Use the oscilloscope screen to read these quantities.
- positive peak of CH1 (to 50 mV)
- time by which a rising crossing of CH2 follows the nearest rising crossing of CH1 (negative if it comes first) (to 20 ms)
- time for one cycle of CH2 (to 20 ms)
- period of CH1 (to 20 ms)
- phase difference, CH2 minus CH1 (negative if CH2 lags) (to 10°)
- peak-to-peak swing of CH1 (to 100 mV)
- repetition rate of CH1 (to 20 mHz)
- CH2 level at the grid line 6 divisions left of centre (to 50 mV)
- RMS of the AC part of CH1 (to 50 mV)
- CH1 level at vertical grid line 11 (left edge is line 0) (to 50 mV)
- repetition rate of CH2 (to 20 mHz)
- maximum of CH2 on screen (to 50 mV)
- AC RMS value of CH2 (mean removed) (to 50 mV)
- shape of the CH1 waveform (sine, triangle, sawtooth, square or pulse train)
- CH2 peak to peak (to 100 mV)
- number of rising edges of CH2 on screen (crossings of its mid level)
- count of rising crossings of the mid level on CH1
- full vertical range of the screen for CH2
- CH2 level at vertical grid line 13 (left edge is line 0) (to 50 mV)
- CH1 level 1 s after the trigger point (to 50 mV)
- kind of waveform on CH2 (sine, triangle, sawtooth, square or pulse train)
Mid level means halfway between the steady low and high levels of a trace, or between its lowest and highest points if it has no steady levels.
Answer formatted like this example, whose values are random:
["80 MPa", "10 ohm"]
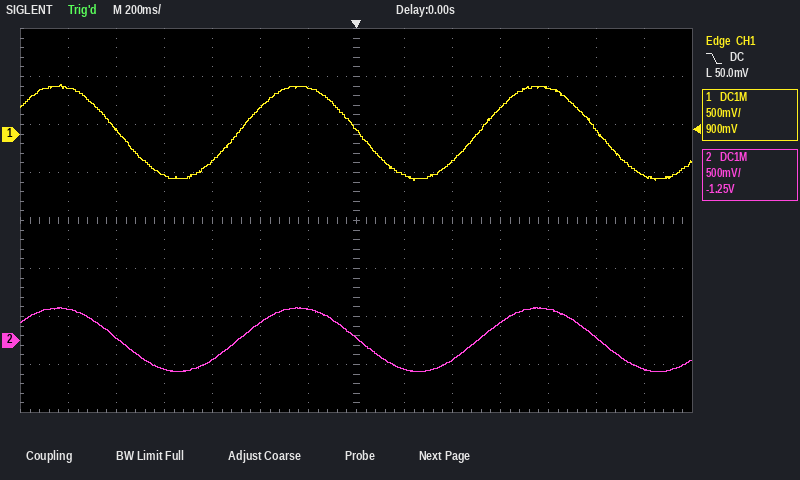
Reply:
["500 mV", "0 ms", "1.00 s", "1.00 s", "0°", "1.00 V", "1.00 Hz", "350 mV", "350 mV", "500 mV", "1.00 Hz", "350 mV", "250 mV", "sine", "700 mV", "2", "2", "4 V", "-300 mV", "50 mV", "sine"]
